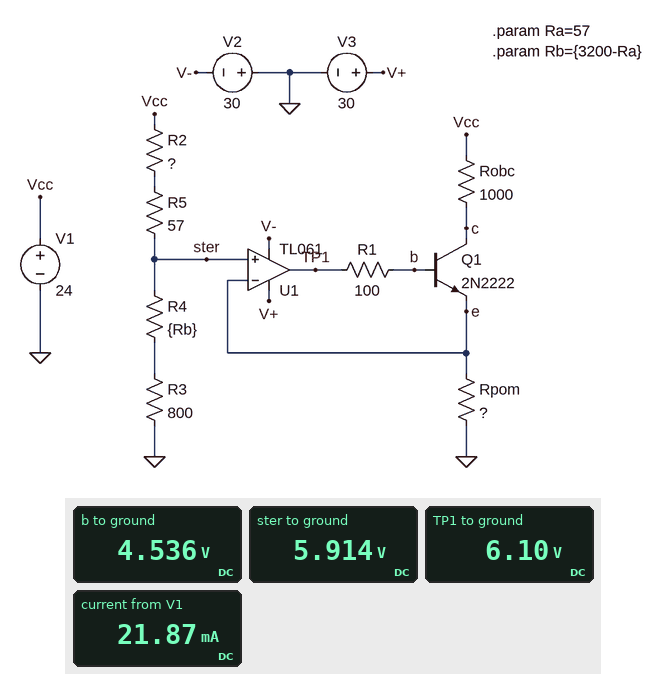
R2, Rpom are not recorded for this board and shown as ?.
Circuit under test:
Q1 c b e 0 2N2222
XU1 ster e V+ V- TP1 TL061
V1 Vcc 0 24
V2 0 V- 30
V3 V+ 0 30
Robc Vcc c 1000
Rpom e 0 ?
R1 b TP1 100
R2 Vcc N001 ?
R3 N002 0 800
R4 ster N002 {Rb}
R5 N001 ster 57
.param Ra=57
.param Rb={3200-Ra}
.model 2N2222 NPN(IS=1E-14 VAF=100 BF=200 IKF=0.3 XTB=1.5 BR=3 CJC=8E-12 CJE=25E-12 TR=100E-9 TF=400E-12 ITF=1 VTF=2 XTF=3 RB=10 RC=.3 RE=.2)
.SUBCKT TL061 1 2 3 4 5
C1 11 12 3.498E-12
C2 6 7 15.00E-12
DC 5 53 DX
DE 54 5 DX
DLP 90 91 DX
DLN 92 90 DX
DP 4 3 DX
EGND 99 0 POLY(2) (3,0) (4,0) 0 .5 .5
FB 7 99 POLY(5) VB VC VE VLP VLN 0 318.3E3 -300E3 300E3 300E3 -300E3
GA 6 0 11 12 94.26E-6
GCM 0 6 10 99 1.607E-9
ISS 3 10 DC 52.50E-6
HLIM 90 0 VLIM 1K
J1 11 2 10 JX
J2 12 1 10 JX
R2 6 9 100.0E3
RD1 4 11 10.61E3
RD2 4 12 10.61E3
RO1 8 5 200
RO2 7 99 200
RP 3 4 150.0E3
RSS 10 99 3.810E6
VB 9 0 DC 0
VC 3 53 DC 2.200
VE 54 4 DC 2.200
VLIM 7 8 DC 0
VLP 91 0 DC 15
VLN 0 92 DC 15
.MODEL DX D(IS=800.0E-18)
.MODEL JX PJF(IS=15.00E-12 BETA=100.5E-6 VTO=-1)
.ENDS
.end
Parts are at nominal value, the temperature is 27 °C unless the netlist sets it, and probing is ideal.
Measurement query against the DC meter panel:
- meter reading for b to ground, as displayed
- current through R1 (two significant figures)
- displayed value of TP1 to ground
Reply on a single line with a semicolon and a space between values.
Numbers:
4.536 V; 16 mA; 6.10 V
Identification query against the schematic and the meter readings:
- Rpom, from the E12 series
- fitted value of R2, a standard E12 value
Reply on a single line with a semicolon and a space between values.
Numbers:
100 Ω; 12 kΩ
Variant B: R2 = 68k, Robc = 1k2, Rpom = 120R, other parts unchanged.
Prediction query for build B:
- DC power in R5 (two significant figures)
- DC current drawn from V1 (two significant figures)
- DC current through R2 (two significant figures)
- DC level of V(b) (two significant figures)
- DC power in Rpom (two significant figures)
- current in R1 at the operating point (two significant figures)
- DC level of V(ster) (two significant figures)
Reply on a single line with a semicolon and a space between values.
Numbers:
6.3 µW; 11 mA; 330 µA; 2.0 V; 14 mW; 52 µA; 1.3 V
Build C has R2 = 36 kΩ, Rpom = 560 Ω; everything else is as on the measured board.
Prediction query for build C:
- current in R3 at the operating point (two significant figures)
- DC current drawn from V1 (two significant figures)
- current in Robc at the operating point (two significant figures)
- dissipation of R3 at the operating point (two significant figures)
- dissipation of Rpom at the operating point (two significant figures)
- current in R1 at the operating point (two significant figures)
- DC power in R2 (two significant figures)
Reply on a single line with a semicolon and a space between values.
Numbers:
600 µA; 4.8 mA; 4.2 mA; 290 µW; 10 mW; 18 µA; 13 mW
